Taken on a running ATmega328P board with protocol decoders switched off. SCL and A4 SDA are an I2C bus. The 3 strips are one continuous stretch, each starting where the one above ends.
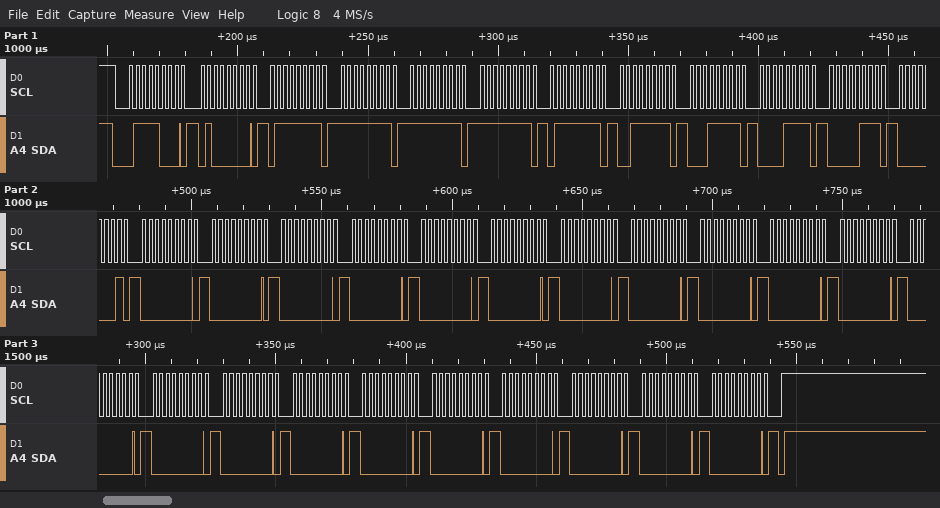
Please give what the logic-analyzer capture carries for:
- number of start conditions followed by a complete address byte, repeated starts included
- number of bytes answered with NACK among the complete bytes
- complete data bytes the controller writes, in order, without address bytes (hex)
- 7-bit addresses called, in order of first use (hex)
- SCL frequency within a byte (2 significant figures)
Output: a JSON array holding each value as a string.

["1", "0", "40 7F FF FF FF 7F 3F 1F 0F 07 01 00 00 00 00 00 00 00 00 00 00 00 00 00 00 00 00 00 00 00 00 00", "0x3C", "400 kHz"]
